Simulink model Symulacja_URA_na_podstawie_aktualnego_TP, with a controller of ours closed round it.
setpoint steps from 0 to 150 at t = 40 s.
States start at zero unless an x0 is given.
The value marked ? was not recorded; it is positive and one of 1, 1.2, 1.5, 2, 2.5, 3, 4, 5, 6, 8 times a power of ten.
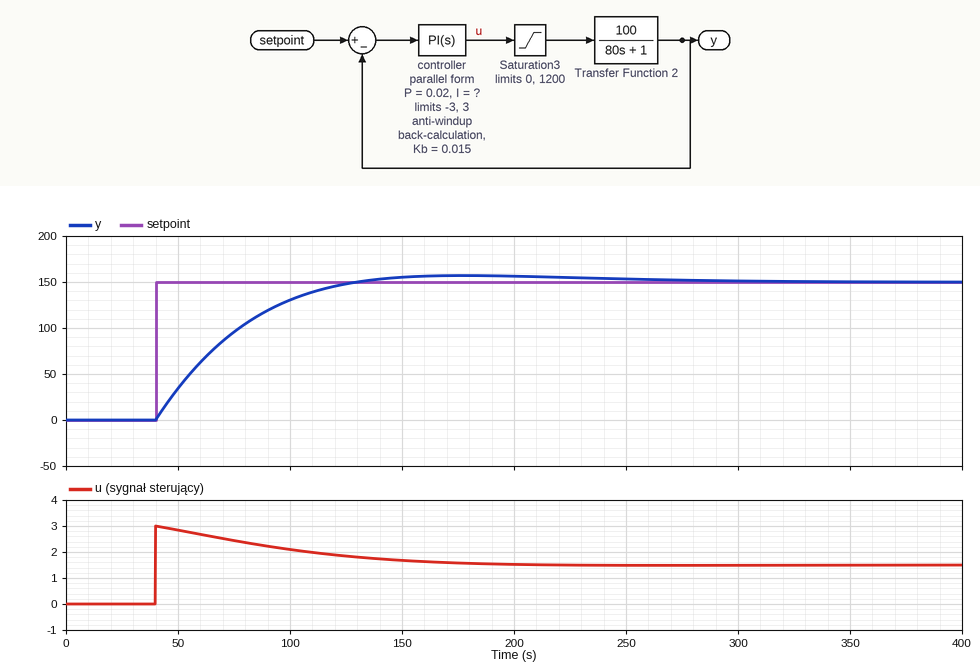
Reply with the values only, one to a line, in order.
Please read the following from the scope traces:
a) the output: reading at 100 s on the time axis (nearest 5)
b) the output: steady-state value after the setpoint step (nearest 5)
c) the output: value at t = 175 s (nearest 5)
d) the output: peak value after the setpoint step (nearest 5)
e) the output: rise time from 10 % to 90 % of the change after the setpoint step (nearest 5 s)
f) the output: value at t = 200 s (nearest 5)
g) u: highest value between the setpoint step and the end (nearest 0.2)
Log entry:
130
150
155
155
60 s
155
3.0
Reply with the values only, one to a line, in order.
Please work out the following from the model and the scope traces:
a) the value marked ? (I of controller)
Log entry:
0.0004
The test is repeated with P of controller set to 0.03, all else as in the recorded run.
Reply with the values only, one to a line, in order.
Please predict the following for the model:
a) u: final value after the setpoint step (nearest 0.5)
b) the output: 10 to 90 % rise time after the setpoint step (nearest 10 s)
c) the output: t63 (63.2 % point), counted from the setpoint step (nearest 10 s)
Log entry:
1.5
60 s
30 s
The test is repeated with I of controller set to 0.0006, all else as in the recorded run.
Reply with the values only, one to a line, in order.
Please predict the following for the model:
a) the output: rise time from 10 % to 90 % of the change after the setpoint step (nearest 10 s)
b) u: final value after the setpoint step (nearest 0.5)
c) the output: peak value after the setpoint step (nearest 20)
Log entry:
50 s
1.5
160
